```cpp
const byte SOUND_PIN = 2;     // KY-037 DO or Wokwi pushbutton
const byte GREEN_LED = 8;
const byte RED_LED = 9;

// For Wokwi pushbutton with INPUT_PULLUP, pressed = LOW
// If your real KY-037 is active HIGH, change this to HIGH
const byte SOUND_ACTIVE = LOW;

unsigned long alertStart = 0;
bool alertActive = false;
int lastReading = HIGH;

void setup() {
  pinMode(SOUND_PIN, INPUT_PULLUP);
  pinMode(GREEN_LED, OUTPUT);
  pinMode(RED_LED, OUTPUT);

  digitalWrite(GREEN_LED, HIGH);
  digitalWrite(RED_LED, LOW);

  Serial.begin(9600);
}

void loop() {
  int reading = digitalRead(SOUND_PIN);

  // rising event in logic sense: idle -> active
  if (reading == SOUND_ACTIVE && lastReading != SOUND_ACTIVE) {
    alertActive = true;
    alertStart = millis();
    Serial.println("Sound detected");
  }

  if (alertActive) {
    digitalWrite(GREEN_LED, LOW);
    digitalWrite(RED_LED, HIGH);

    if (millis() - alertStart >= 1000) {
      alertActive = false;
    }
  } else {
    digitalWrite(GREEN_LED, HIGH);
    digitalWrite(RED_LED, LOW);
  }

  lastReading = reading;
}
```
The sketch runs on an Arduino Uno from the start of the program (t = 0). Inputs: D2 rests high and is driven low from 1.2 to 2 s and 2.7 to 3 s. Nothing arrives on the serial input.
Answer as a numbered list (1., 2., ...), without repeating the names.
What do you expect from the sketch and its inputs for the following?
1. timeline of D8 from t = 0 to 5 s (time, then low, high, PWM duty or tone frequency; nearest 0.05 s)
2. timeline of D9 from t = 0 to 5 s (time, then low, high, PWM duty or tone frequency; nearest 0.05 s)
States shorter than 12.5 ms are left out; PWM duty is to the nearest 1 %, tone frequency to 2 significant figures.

1. 0 s high; 1.2 s low; 2.2 s high; 2.7 s low; 3.7 s high
2. 0 s low; 1.2 s high; 2.2 s low; 2.7 s high; 3.7 s low
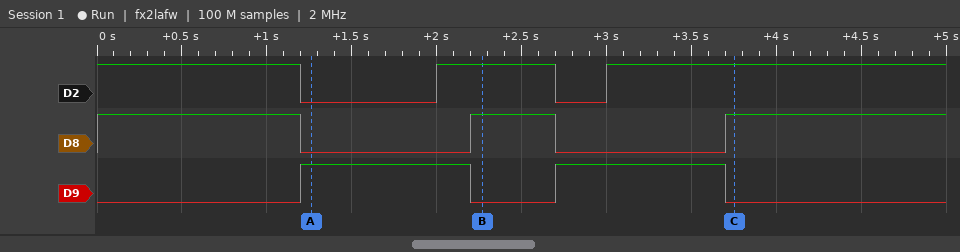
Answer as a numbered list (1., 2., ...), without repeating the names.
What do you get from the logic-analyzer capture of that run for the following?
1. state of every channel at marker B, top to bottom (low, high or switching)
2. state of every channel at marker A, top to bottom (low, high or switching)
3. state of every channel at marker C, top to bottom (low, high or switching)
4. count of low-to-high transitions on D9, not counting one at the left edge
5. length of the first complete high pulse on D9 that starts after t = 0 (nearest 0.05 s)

1. D2 high, D8 high, D9 low
2. D2 low, D8 low, D9 high
3. D2 high, D8 high, D9 low
4. 2
5. 1.00 s
